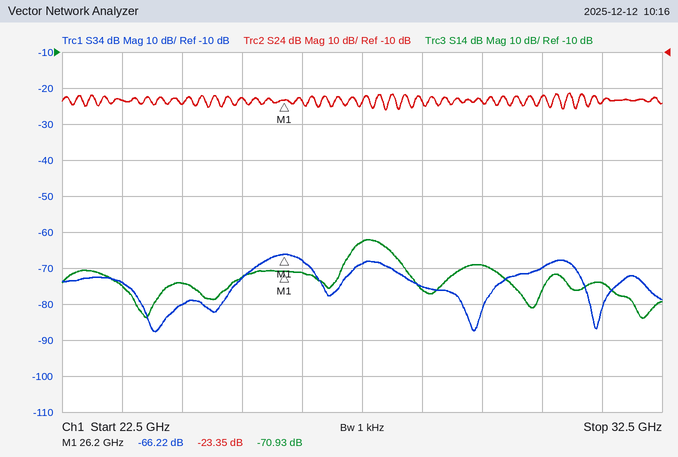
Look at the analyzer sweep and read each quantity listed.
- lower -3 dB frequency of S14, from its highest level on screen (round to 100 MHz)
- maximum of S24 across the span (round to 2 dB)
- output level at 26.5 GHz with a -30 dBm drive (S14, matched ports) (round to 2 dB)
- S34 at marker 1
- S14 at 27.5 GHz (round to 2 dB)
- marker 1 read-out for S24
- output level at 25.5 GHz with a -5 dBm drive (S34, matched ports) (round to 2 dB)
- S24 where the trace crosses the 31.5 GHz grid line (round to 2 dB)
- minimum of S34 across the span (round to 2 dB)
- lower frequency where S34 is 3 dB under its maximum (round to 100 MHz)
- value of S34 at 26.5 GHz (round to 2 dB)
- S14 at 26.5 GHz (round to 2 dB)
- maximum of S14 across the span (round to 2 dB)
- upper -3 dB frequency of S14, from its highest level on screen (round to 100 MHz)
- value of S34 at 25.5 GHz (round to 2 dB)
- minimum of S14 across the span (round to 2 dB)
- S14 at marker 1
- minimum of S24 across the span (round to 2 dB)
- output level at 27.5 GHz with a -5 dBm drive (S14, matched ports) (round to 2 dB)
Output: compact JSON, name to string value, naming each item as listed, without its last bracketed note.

{"lower -3 dB frequency of S14, from its highest level on screen": "27.3 GHz", "maximum of S24 across the span": "-22 dB", "output level at 26.5 GHz with a -30 dBm drive (S14, matched ports)": "-102 dBm", "S34 at marker 1": "-66.22 dB", "S14 at 27.5 GHz": "-62 dB", "marker 1 read-out for S24": "-23.35 dB", "output level at 25.5 GHz with a -5 dBm drive (S34, matched ports)": "-78 dBm", "S24 where the trace crosses the 31.5 GHz grid line": "-24 dB", "minimum of S34 across the span": "-88 dB", "lower frequency where S34 is 3 dB under its maximum": "25.8 GHz", "value of S34 at 26.5 GHz": "-68 dB", "S14 at 26.5 GHz": "-72 dB", "maximum of S14 across the span": "-62 dB", "upper -3 dB frequency of S14, from its highest level on screen": "28.0 GHz", "value of S34 at 25.5 GHz": "-72 dB", "minimum of S14 across the span": "-84 dB", "S14 at marker 1": "-70.93 dB", "minimum of S24 across the span": "-26 dB", "output level at 27.5 GHz with a -5 dBm drive (S14, matched ports)": "-68 dBm"}
